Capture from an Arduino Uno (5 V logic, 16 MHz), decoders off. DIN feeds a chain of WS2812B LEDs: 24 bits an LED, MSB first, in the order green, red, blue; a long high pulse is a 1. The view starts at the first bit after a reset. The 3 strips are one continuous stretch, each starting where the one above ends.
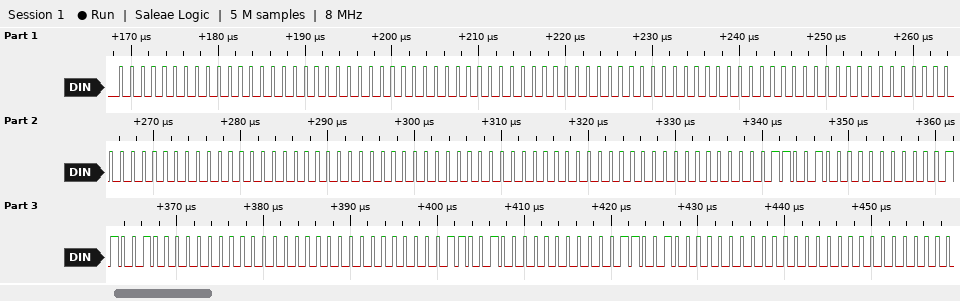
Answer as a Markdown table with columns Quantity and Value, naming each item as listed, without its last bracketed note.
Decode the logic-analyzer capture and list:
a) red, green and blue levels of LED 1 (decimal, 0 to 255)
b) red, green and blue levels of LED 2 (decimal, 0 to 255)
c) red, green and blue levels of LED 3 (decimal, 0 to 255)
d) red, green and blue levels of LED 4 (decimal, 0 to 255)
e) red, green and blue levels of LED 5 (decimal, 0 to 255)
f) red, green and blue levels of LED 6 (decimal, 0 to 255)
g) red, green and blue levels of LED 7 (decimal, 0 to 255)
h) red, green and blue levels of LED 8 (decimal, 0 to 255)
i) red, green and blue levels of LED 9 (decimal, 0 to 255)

| Quantity | Value |
|---|---|
| red, green and blue levels of LED 1 | 0, 0, 0 |
| red, green and blue levels of LED 2 | 0, 0, 0 |
| red, green and blue levels of LED 3 | 0, 0, 0 |
| red, green and blue levels of LED 4 | 0, 0, 0 |
| red, green and blue levels of LED 5 | 0, 0, 0 |
| red, green and blue levels of LED 6 | 0, 0, 50 |
| red, green and blue levels of LED 7 | 50, 0, 0 |
| red, green and blue levels of LED 8 | 0, 0, 50 |
| red, green and blue levels of LED 9 | 50, 0, 0 |
